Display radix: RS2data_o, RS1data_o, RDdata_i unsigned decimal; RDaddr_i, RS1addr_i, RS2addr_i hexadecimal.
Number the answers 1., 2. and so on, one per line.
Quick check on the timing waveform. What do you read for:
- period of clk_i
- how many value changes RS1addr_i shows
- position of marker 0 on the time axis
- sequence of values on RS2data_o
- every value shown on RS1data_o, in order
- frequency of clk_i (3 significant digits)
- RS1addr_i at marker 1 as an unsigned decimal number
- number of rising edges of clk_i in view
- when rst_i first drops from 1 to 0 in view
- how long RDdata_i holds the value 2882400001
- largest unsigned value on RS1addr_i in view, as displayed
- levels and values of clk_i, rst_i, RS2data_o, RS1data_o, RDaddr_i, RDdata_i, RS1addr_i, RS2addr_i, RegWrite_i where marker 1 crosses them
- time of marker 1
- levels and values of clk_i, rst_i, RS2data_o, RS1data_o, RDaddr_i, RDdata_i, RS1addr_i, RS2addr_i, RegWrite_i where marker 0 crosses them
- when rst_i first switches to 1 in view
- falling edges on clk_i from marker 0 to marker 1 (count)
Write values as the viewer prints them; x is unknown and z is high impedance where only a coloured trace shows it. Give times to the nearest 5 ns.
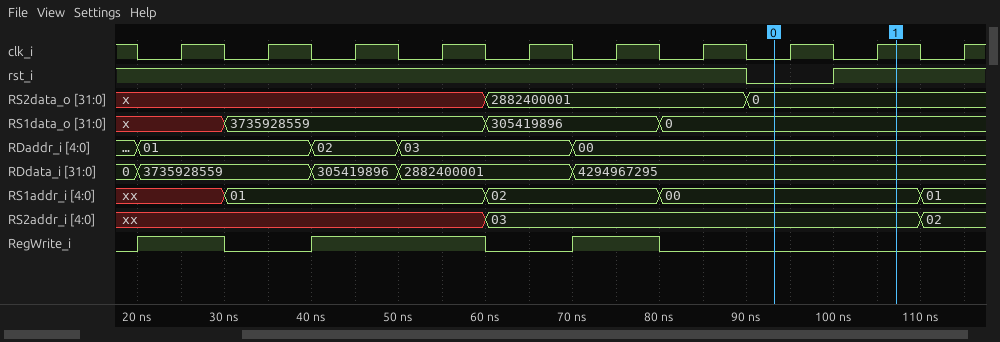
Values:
1. 10 ns
2. 4
3. 95 ns
4. x, 2882400001, 0
5. x, 3735928559, 305419896, 0
6. 100 MHz
7. 0
8. 10
9. 90 ns
10. 20 ns
11. 02
12. clk_i=1, rst_i=1, RS2data_o=0, RS1data_o=0, RDaddr_i=00, RDdata_i=4294967295, RS1addr_i=00, RS2addr_i=03, RegWrite_i=0
13. 105 ns
14. clk_i=0, rst_i=0, RS2data_o=0, RS1data_o=0, RDaddr_i=00, RDdata_i=4294967295, RS1addr_i=00, RS2addr_i=03, RegWrite_i=0
15. 100 ns
16. 1
